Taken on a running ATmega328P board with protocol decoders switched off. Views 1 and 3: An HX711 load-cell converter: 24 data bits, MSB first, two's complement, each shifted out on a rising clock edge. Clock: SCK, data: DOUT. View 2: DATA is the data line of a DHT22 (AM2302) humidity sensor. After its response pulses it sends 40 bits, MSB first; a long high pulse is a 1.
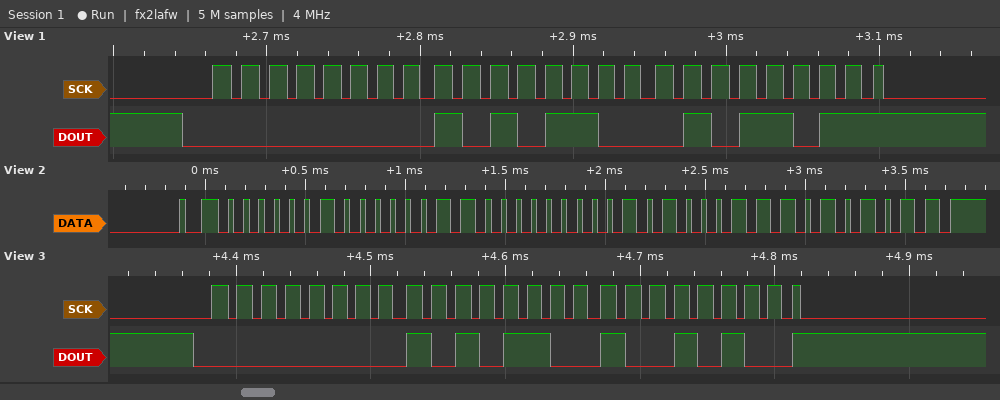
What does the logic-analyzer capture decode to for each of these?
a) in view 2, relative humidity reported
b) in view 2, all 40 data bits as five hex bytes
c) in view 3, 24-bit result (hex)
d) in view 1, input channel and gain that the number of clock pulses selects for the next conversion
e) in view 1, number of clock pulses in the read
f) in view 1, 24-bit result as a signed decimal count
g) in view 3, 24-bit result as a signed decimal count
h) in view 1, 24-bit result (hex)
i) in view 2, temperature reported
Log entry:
51.8 %
02 06 00 A3 AB
0x00AC94
channel A, gain 128
25
44123
44180
0x00AC5B
16.3 °C
